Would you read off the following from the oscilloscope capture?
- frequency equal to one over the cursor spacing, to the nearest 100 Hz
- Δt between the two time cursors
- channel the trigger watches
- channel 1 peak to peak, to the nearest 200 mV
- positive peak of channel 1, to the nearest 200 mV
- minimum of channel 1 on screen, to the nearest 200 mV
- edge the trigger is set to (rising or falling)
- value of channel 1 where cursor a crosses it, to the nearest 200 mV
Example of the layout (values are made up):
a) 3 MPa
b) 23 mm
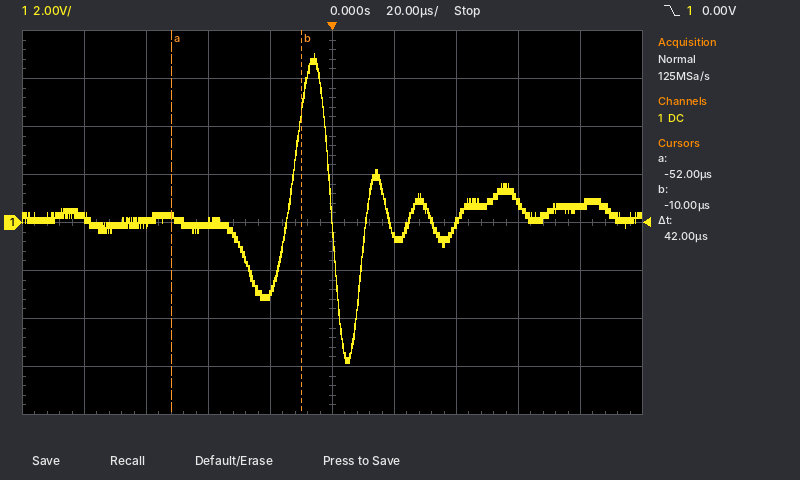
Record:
a) 23.8 kHz
b) 42 µs
c) channel 1
d) 12.8 V
e) 7.0 V
f) -5.8 V
g) falling
h) 200 mV
